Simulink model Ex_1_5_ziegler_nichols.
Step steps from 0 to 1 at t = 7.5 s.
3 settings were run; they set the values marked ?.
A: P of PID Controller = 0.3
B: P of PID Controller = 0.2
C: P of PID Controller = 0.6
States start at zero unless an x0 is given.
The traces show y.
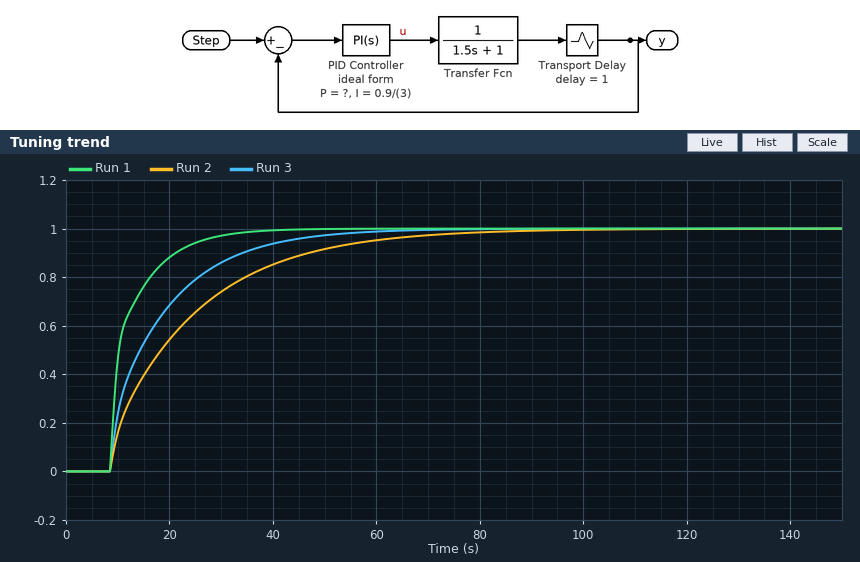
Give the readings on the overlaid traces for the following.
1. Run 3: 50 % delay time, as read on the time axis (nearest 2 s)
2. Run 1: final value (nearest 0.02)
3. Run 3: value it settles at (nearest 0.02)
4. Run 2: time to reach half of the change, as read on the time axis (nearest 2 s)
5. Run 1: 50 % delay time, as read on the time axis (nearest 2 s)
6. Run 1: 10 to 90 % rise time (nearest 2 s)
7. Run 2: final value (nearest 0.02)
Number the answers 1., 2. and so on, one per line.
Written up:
1. 14 s
2. 1.00
3. 1.00
4. 18 s
5. 10 s
6. 12 s
7. 1.00
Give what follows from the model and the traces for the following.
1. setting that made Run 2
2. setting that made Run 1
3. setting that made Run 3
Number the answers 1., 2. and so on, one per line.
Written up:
1. B
2. C
3. A
